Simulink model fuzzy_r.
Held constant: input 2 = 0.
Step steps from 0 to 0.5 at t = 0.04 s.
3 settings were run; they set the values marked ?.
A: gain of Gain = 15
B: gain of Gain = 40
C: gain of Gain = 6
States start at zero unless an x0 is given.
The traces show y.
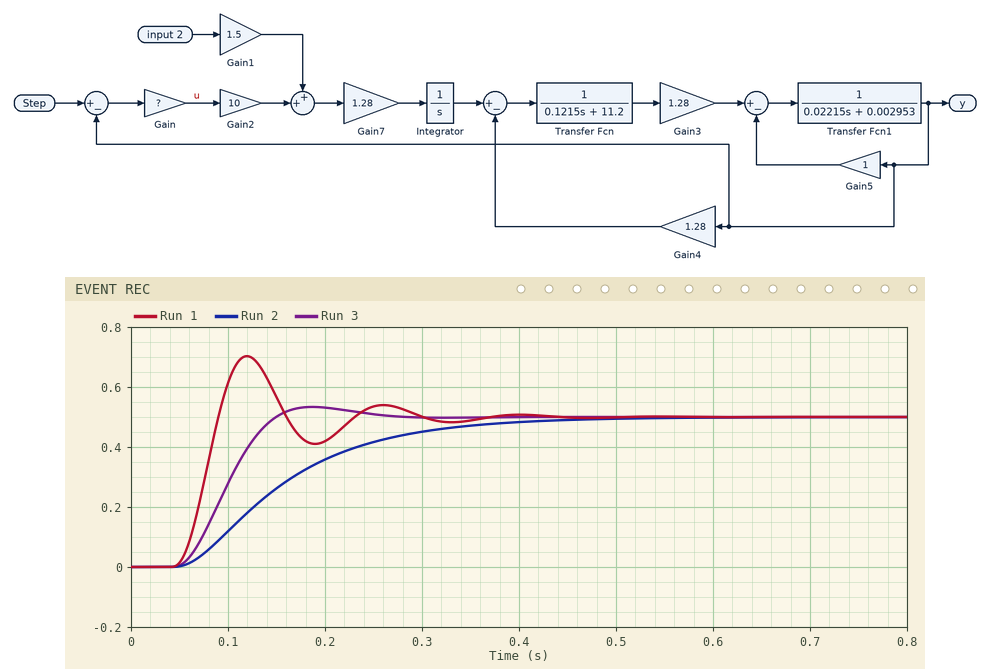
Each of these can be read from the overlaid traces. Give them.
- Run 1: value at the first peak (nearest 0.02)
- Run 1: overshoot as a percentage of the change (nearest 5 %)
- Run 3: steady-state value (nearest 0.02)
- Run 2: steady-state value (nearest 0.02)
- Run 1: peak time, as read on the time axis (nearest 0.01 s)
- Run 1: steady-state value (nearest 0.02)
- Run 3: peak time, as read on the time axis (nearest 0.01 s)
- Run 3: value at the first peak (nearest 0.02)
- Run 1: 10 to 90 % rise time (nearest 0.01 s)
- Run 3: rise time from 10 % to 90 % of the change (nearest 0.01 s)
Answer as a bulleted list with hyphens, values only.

- 0.70
- 40 %
- 0.50
- 0.50
- 0.12 s
- 0.50
- 0.19 s
- 0.54
- 0.03 s
- 0.07 s
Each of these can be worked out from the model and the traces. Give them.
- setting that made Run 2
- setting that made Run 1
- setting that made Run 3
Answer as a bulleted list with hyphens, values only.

- C
- B
- A
